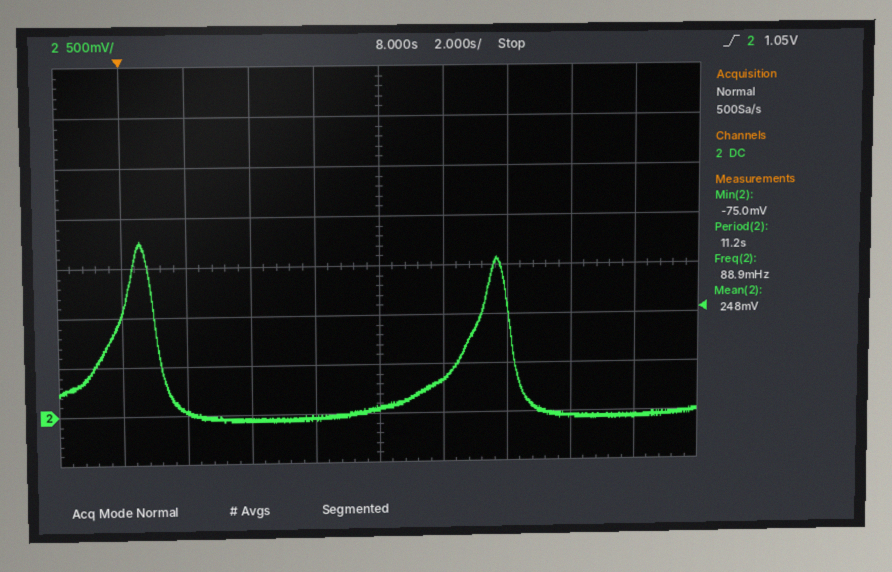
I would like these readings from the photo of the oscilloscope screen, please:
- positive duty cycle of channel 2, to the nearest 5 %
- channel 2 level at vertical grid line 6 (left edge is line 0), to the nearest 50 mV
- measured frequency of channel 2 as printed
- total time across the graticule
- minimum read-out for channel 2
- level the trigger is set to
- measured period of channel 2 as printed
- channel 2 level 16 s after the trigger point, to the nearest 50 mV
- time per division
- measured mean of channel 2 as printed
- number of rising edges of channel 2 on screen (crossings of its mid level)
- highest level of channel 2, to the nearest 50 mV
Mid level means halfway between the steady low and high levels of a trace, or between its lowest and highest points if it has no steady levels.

10 %
350 mV
88.9 mHz
20 s
-75.0 mV
1.05 V
11.2 s
-50 mV
2 s
248 mV
2
1.75 V
